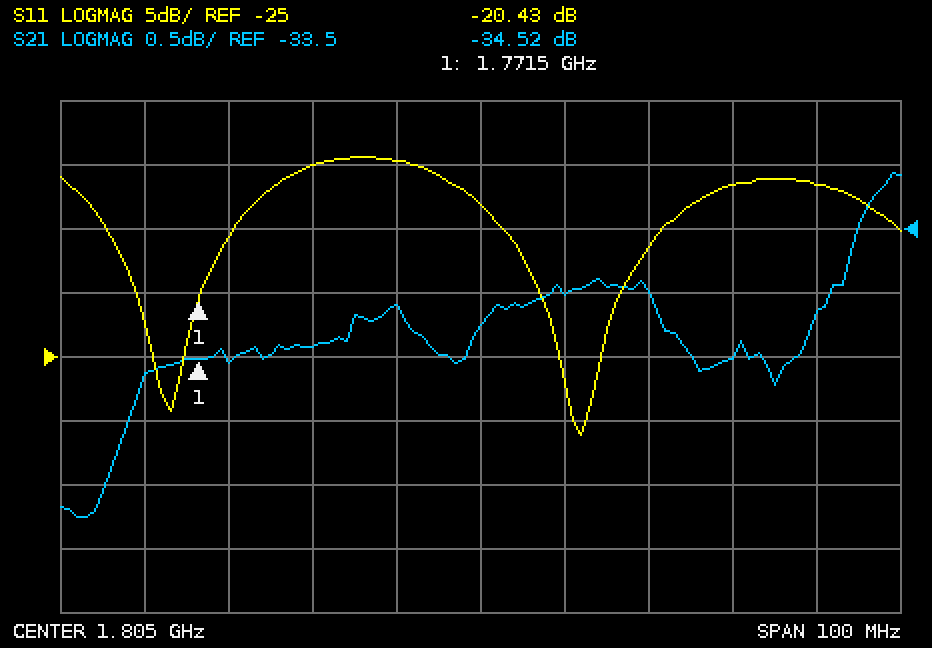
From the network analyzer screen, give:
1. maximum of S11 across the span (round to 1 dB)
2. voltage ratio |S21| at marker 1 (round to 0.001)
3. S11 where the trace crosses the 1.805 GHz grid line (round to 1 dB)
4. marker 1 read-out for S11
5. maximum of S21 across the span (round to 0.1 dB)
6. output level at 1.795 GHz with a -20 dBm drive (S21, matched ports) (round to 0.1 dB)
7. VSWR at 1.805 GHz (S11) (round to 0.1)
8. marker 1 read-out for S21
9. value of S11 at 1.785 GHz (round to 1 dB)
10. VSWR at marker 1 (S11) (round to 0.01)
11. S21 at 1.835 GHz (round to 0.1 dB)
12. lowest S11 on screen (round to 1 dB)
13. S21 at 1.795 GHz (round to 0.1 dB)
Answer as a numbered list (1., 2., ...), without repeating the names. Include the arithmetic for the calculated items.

1. -9 dB
2. 10^(-34.52/20) ≈ 0.019
3. -13 dB
4. -20.43 dB
5. -33.1 dB
6. -20 dBm + (-34.1 dB) = -54.1 dBm
7. |Γ| = 10^(-13/20) = 0.2239; VSWR = (1 + 0.2239)/(1 − 0.2239) ≈ 1.6
8. -34.52 dB
9. -10 dB
10. (1 + 0.0952)/(1 − 0.0952) ≈ 1.21
11. -34.5 dB
12. -31 dB
13. -34.1 dB
